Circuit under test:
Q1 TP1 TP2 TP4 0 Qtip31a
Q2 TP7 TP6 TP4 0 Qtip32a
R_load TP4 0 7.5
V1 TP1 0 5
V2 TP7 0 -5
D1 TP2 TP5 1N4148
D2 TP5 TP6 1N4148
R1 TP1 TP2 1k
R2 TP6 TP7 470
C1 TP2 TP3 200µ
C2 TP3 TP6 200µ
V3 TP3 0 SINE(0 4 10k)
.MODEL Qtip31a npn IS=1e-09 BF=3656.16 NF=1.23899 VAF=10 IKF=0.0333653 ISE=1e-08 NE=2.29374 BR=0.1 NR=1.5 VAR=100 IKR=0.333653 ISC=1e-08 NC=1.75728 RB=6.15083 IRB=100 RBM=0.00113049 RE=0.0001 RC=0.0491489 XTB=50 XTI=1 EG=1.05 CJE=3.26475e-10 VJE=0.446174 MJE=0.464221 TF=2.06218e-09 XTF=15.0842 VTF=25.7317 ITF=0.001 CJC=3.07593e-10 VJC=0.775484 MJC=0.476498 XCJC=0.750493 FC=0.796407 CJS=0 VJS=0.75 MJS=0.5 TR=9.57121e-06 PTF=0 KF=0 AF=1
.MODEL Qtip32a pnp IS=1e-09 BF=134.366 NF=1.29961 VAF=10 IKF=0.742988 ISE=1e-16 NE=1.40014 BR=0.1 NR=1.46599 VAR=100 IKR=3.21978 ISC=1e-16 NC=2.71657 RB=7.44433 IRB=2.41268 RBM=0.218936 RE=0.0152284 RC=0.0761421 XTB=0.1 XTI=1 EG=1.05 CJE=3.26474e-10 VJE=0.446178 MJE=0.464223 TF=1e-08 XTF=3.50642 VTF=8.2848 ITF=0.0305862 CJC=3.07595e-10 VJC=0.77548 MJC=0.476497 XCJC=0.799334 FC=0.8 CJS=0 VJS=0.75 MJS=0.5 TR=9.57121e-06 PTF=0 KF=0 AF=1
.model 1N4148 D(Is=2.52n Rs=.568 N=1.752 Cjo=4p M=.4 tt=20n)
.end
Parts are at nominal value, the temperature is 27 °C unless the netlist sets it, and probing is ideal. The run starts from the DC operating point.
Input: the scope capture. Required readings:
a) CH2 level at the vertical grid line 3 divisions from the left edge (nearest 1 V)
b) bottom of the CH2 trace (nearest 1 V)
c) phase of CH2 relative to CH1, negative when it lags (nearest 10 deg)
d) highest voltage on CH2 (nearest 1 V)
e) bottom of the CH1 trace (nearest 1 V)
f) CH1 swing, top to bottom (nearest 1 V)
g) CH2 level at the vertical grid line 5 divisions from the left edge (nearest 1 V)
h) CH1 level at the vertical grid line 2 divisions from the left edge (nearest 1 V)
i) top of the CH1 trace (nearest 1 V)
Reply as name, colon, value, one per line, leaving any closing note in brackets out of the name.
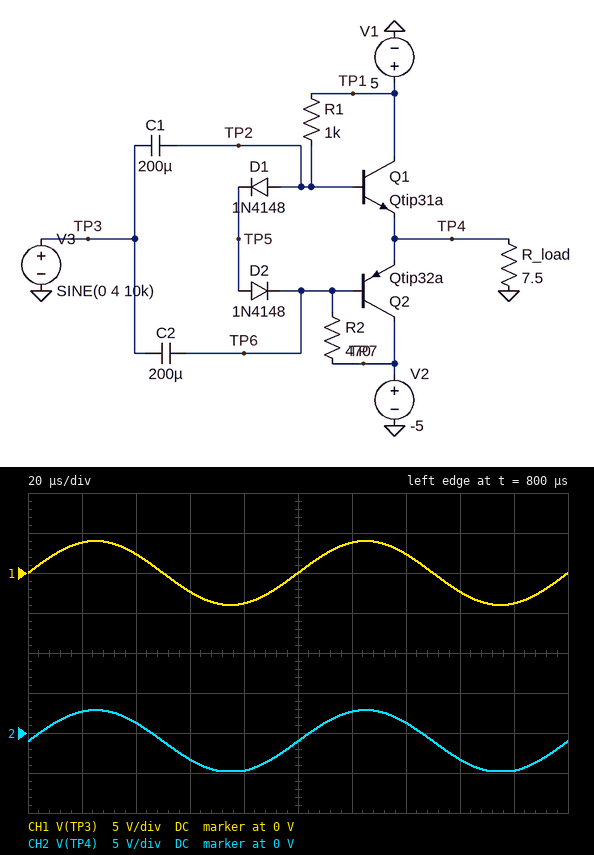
CH2 level at the vertical grid line 3 divisions from the left edge: -3 V
bottom of the CH2 trace: -5 V
phase of CH2 relative to CH1, negative when it lags: 0 deg
highest voltage on CH2: 3 V
bottom of the CH1 trace: -4 V
CH1 swing, top to bottom: 8 V
CH2 level at the vertical grid line 5 divisions from the left edge: -1 V
CH1 level at the vertical grid line 2 divisions from the left edge: 2 V
top of the CH1 trace: 4 V
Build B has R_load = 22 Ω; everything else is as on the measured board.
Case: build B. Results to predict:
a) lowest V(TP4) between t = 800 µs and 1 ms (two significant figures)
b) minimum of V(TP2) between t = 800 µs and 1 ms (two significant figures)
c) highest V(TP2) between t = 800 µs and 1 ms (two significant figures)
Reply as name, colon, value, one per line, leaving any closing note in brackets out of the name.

lowest V(TP4) between t = 800 µs and 1 ms: -4.9 V
minimum of V(TP2) between t = 800 µs and 1 ms: -4.6 V
highest V(TP2) between t = 800 µs and 1 ms: 3.4 V
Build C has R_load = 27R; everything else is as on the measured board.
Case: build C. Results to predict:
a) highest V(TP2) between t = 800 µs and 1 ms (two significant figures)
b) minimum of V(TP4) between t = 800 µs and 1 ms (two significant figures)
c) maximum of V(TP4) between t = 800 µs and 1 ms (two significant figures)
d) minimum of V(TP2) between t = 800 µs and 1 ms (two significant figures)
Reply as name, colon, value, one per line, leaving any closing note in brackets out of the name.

highest V(TP2) between t = 800 µs and 1 ms: 3.4 V
minimum of V(TP4) between t = 800 µs and 1 ms: -4.9 V
maximum of V(TP4) between t = 800 µs and 1 ms: 2.7 V
minimum of V(TP2) between t = 800 µs and 1 ms: -4.6 V
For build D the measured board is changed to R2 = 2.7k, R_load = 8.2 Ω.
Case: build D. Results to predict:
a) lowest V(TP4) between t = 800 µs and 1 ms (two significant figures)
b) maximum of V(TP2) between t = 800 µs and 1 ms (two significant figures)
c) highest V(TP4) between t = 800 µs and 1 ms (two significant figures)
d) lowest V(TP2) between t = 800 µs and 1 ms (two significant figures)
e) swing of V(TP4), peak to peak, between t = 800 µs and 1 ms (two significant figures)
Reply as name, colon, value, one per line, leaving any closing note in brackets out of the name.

lowest V(TP4) between t = 800 µs and 1 ms: -2.5 V
maximum of V(TP2) between t = 800 µs and 1 ms: 6.0 V
highest V(TP4) between t = 800 µs and 1 ms: 4.8 V
lowest V(TP2) between t = 800 µs and 1 ms: -2.0 V
swing of V(TP4), peak to peak, between t = 800 µs and 1 ms: 7.3 V
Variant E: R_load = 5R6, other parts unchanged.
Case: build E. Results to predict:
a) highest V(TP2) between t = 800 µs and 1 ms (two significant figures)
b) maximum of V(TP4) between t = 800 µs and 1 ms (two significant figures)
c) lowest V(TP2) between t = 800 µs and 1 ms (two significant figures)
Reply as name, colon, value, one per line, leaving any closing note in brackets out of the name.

highest V(TP2) between t = 800 µs and 1 ms: 3.7 V
maximum of V(TP4) between t = 800 µs and 1 ms: 2.9 V
lowest V(TP2) between t = 800 µs and 1 ms: -4.3 V
